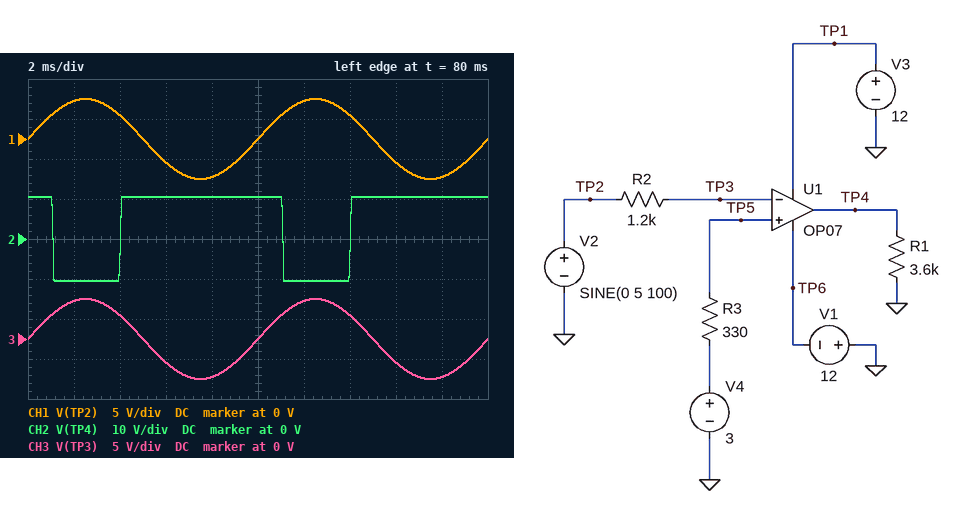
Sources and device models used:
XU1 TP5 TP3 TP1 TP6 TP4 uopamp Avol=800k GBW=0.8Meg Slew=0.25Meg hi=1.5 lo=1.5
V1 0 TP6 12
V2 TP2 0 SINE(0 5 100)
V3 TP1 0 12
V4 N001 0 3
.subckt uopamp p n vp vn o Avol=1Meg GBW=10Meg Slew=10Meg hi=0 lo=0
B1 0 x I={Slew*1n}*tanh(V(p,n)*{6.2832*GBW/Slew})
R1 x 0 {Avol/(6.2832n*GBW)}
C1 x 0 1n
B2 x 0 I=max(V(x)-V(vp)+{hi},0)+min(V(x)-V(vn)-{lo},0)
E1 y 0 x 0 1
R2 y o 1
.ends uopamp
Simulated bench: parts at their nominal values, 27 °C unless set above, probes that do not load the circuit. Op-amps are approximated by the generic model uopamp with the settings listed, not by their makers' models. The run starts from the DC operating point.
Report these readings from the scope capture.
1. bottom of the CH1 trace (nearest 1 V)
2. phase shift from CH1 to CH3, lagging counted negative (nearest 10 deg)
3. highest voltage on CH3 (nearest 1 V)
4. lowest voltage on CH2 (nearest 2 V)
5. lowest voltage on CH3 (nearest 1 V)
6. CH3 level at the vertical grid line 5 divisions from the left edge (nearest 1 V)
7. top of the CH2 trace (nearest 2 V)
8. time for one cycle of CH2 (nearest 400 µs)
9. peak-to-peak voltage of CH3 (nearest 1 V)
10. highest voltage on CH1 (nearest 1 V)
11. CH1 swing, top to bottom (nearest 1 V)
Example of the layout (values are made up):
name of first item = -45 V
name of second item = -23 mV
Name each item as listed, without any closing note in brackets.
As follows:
bottom of the CH1 trace = -5 V
phase shift from CH1 to CH3, lagging counted negative = 0 deg
highest voltage on CH3 = 5 V
lowest voltage on CH2 = -10 V
lowest voltage on CH3 = -5 V
CH3 level at the vertical grid line 5 divisions from the left edge = 0 V
top of the CH2 trace = 10 V
time for one cycle of CH2 = 10.0 ms
peak-to-peak voltage of CH3 = 10 V
highest voltage on CH1 = 5 V
CH1 swing, top to bottom = 10 V
